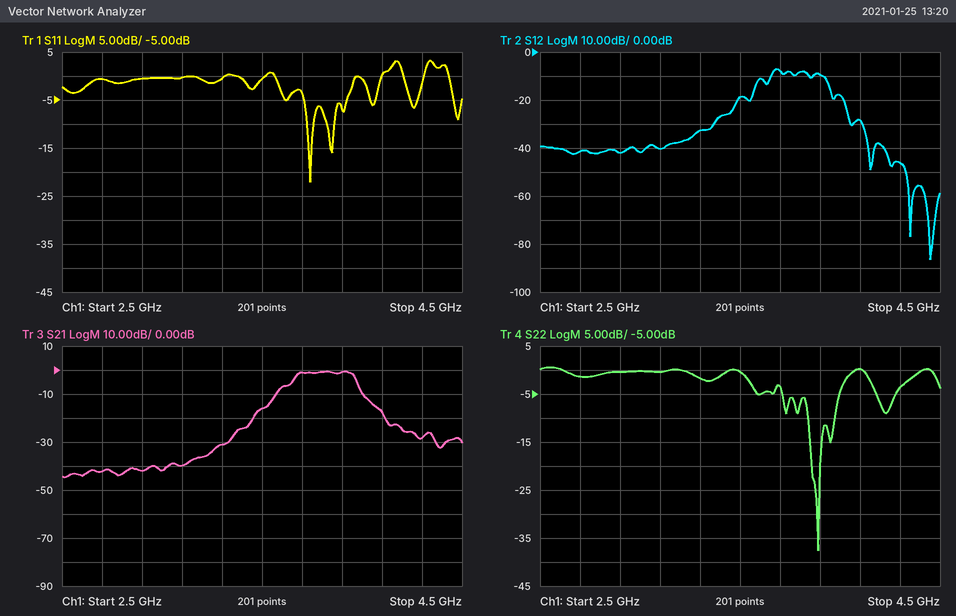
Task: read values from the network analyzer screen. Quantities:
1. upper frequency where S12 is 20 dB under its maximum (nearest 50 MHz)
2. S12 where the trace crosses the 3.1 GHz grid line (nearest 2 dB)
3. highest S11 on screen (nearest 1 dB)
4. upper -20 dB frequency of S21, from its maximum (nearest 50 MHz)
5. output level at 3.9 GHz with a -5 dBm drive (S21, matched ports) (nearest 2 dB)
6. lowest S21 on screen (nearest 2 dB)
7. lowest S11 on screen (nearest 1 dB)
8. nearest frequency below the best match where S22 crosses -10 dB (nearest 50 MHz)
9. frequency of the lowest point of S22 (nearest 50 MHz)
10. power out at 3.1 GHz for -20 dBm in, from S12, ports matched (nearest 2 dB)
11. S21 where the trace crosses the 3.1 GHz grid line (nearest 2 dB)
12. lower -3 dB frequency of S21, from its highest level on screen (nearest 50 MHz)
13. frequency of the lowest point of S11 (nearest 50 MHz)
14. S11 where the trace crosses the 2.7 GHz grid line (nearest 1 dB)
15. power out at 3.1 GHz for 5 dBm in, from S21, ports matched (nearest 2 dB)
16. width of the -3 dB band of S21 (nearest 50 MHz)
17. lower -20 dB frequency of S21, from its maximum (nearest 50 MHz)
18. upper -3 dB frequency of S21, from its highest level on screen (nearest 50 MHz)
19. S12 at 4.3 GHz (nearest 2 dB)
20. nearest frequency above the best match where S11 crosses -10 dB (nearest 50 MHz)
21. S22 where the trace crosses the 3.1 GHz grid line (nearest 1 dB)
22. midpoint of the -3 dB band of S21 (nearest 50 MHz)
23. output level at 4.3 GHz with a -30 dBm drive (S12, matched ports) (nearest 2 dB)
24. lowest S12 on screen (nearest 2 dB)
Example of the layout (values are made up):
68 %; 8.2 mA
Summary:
4.05 GHz; -40 dB; 3 dB; 4.10 GHz; -6 dBm; -44 dB; -22 dB; 3.85 GHz; 3.90 GHz; -60 dBm; -40 dB; 3.65 GHz; 3.75 GHz; -1 dB; -34 dBm; 300 MHz; 3.45 GHz; 3.95 GHz; -46 dB; 3.75 GHz; 0 dB; 3.80 GHz; -76 dBm; -86 dB
